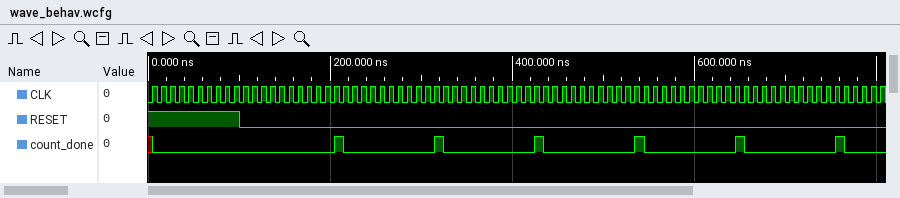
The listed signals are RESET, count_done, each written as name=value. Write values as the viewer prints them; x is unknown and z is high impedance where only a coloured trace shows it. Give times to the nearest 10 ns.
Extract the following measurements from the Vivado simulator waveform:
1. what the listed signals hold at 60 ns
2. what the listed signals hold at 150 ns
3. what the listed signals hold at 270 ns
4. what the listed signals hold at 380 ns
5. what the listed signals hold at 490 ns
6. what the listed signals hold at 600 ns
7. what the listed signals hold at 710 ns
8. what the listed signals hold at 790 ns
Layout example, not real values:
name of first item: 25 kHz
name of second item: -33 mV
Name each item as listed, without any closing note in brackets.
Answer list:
what the listed signals hold at 60 ns: RESET=1, count_done=0
what the listed signals hold at 150 ns: RESET=0, count_done=0
what the listed signals hold at 270 ns: RESET=0, count_done=0
what the listed signals hold at 380 ns: RESET=0, count_done=0
what the listed signals hold at 490 ns: RESET=0, count_done=0
what the listed signals hold at 600 ns: RESET=0, count_done=0
what the listed signals hold at 710 ns: RESET=0, count_done=0
what the listed signals hold at 790 ns: RESET=0, count_done=0
